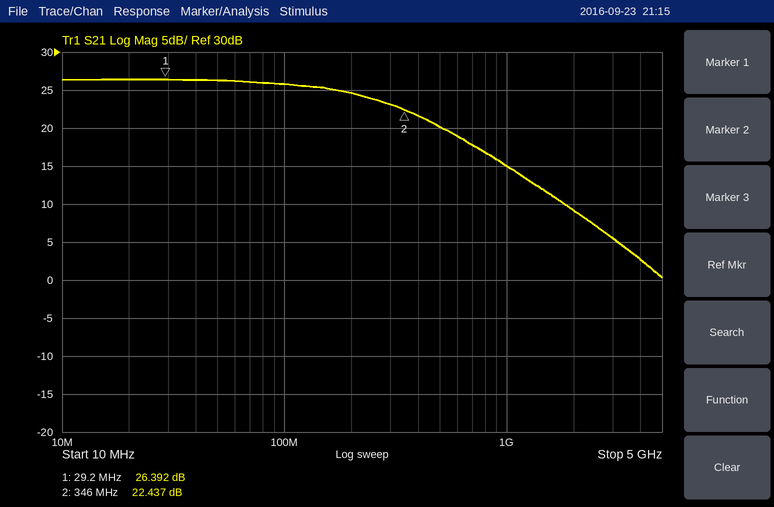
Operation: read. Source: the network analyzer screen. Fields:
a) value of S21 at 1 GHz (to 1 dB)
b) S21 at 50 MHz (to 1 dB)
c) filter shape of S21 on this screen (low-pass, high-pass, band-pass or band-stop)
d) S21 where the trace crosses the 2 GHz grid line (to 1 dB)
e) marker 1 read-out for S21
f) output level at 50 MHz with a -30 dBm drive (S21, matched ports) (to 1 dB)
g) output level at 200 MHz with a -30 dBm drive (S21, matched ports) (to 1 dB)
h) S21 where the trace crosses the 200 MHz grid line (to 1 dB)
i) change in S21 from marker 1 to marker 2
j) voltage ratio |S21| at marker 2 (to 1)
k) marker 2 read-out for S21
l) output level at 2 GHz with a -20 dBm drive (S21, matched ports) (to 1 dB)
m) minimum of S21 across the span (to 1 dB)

15 dB
26 dB
low-pass
9 dB
26.392 dB
-4 dBm
-5 dBm
25 dB
-3.955 dB
13
22.437 dB
-11 dBm
0 dB
